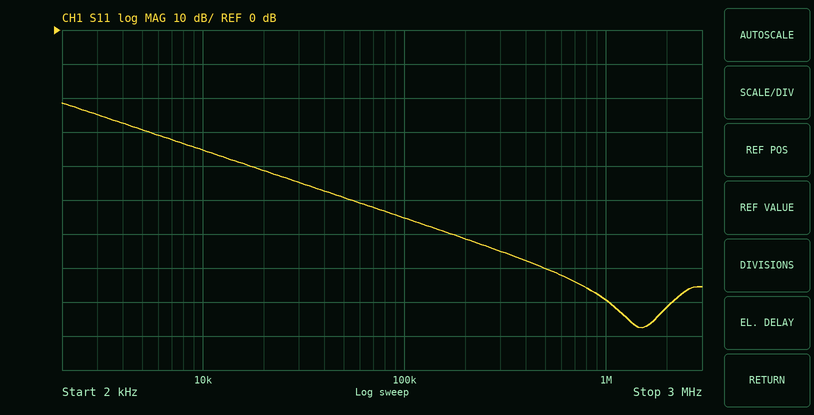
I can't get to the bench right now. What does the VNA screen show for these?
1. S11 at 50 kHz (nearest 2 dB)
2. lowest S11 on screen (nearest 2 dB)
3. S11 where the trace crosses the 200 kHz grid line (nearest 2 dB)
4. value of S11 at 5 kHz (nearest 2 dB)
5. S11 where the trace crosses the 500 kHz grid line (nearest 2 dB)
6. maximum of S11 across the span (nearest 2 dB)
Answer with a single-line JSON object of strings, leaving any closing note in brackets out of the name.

{"S11 at 50 kHz": "-50 dB", "lowest S11 on screen": "-88 dB", "S11 where the trace crosses the 200 kHz grid line": "-62 dB", "value of S11 at 5 kHz": "-30 dB", "S11 where the trace crosses the 500 kHz grid line": "-70 dB", "maximum of S11 across the span": "-22 dB"}
